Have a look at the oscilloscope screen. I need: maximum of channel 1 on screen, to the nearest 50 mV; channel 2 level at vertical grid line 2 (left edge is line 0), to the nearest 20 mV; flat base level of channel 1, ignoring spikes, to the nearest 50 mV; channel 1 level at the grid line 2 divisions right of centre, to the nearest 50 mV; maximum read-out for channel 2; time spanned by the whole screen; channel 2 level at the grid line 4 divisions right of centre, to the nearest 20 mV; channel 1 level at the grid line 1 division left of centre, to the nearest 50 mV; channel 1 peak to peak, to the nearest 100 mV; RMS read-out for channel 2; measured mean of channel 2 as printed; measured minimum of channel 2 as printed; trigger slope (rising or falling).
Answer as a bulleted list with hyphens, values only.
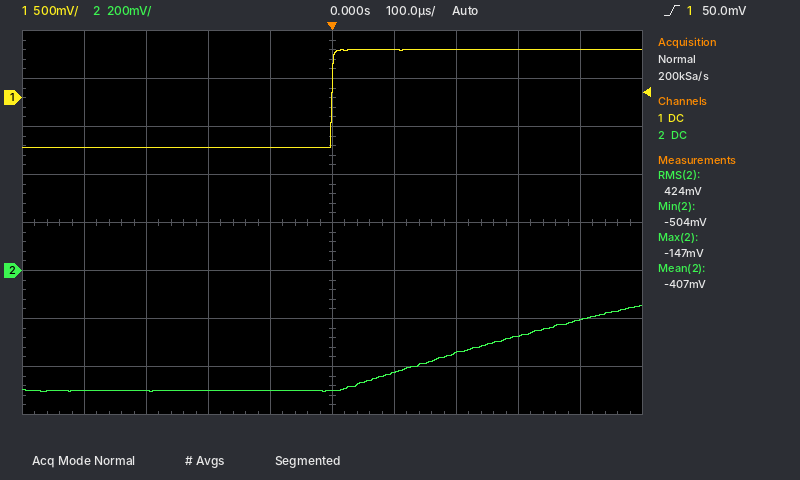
- 500 mV
- -500 mV
- -500 mV
- 500 mV
- -147 mV
- 1 ms
- -200 mV
- -500 mV
- 1.00 V
- 424 mV
- -407 mV
- -504 mV
- rising
